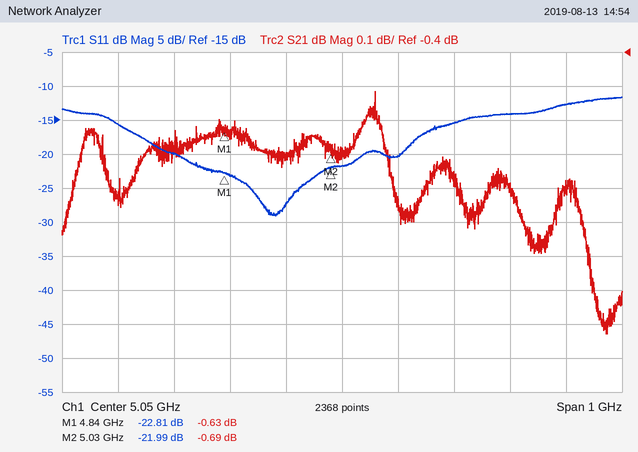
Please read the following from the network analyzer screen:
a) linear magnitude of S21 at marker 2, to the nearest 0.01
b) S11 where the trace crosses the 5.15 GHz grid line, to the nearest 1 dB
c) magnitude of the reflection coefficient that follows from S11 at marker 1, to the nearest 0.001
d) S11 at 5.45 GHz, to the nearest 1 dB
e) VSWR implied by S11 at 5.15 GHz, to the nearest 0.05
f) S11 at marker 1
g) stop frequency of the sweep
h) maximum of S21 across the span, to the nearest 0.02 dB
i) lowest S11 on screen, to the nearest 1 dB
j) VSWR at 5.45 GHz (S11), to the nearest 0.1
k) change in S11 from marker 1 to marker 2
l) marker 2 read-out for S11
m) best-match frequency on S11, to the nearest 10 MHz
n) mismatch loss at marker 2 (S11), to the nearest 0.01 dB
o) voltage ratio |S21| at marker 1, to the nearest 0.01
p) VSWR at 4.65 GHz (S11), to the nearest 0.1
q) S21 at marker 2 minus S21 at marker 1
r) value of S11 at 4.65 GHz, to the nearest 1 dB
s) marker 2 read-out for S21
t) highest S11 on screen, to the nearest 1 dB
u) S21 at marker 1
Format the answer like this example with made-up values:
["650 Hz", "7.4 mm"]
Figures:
["0.92", "-20 dB", "0.072", "-13 dB", "1.20", "-22.81 dB", "5.55 GHz", "-0.52 dB", "-29 dB", "1.6", "0.82 dB", "-21.99 dB", "4.93 GHz", "0.03 dB", "0.93", "1.4", "-0.06 dB", "-16 dB", "-0.69 dB", "-12 dB", "-0.63 dB"]
